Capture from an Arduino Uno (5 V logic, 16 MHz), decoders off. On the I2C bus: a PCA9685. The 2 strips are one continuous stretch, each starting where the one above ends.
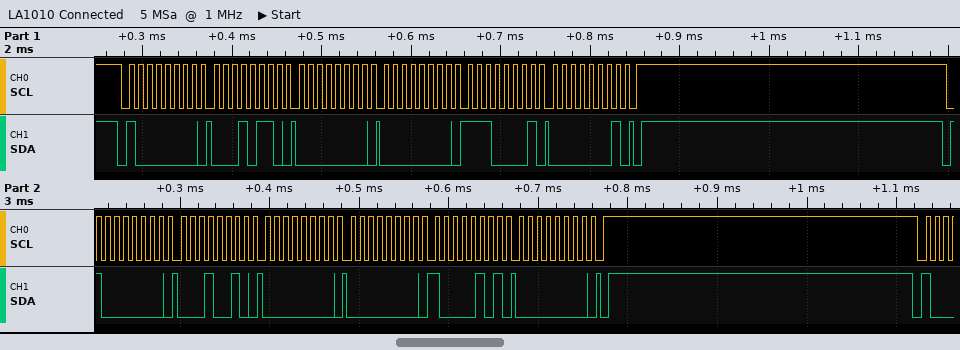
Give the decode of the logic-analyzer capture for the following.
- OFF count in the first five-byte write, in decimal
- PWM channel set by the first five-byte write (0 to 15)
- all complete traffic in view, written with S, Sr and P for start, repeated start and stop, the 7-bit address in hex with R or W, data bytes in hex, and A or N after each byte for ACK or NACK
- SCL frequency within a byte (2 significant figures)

481
4
S 40W A 16 A 00 A 00 A E1 A 01 A P S 40W A 12 A 00 A 00 A 85 A 00 A P
100 kHz
